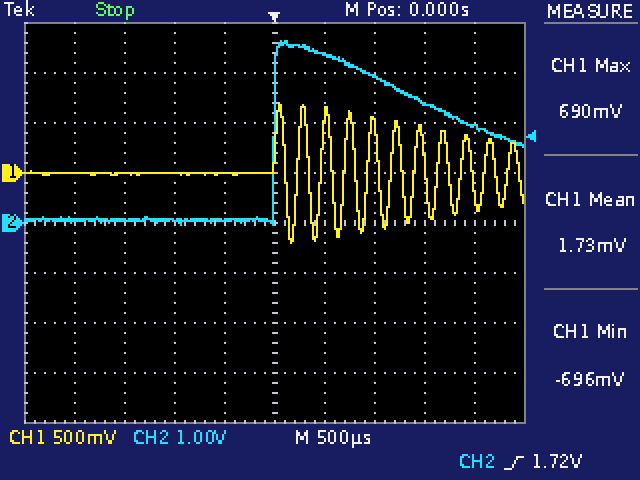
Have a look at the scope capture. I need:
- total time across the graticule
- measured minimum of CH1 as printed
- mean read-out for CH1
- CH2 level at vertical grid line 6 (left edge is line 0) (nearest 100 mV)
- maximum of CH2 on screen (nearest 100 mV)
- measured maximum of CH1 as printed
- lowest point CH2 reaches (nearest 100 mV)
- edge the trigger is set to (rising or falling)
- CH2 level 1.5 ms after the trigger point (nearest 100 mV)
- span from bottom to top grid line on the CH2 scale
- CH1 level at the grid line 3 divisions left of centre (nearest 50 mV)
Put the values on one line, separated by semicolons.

5 ms; -696 mV; 1.73 mV; 3.4 V; 3.6 V; 690 mV; 0.0 V; rising; 2.4 V; 8 V; 0 mV
